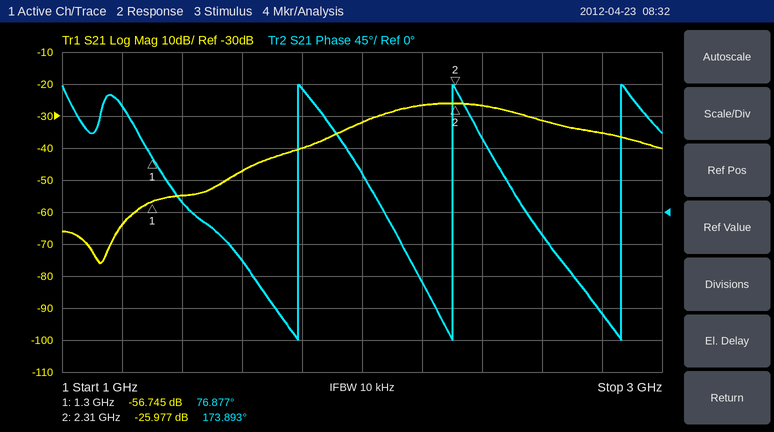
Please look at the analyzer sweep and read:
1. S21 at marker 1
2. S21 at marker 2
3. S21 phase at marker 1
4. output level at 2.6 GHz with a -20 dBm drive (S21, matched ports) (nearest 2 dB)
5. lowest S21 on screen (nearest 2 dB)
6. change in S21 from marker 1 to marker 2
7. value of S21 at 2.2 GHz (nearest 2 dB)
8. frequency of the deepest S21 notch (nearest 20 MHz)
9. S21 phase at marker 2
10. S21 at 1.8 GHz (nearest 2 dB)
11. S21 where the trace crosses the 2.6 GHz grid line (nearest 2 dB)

-56.745 dB
-25.977 dB
76.877°
-52 dBm
-76 dB
30.768 dB
-26 dB
1.12 GHz
173.893°
-40 dB
-32 dB
